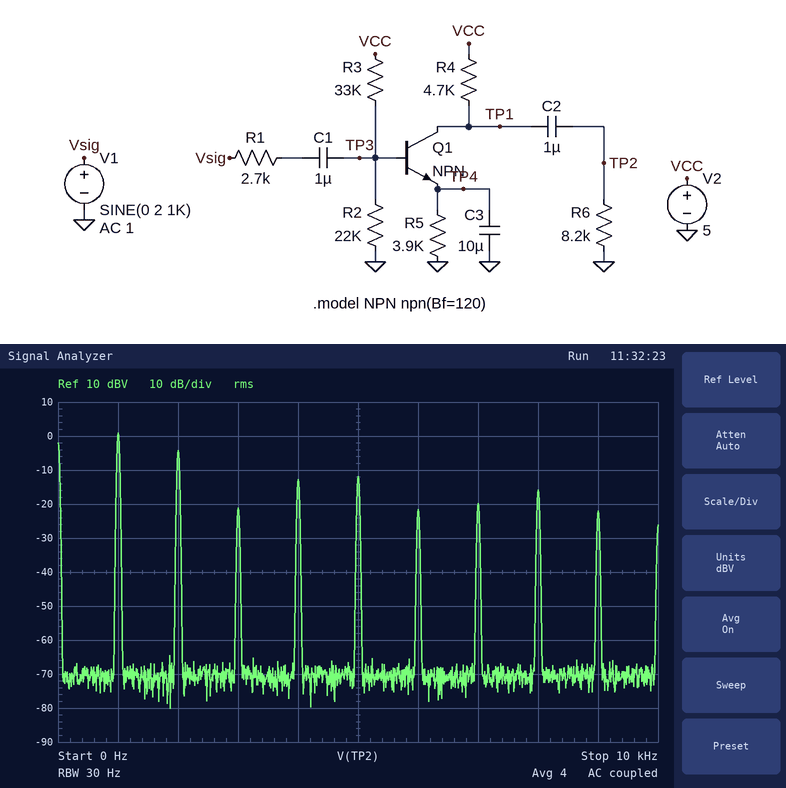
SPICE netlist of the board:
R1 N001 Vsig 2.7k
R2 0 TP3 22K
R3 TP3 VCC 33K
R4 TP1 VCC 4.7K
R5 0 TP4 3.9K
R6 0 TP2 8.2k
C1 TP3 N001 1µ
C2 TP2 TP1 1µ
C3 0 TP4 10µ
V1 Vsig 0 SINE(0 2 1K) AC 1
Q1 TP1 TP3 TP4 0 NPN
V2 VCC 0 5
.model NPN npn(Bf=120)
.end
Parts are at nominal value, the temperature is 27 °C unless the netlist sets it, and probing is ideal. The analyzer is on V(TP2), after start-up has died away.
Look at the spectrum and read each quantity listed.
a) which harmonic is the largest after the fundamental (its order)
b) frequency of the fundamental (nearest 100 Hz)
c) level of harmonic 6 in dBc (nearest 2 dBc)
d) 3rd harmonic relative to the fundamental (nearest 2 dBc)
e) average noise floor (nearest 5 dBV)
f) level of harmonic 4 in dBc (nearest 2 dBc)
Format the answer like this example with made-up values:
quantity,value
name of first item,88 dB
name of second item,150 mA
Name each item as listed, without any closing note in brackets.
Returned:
quantity,value
which harmonic is the largest after the fundamental,2
frequency of the fundamental,1.0 kHz
level of harmonic 6 in dBc,-22 dBc
3rd harmonic relative to the fundamental,-22 dBc
average noise floor,-70 dBV
level of harmonic 4 in dBc,-14 dBc
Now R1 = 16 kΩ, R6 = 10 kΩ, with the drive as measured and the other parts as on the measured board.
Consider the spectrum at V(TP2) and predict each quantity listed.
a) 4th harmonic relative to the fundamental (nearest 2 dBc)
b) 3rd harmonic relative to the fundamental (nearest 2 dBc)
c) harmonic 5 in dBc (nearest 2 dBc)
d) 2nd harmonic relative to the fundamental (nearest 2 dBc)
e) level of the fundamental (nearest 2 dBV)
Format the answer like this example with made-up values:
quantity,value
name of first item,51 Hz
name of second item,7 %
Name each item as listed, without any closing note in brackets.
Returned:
quantity,value
4th harmonic relative to the fundamental,-12 dBc
3rd harmonic relative to the fundamental,-16 dBc
harmonic 5 in dBc,-24 dBc
2nd harmonic relative to the fundamental,-8 dBc
level of the fundamental,2 dBV
